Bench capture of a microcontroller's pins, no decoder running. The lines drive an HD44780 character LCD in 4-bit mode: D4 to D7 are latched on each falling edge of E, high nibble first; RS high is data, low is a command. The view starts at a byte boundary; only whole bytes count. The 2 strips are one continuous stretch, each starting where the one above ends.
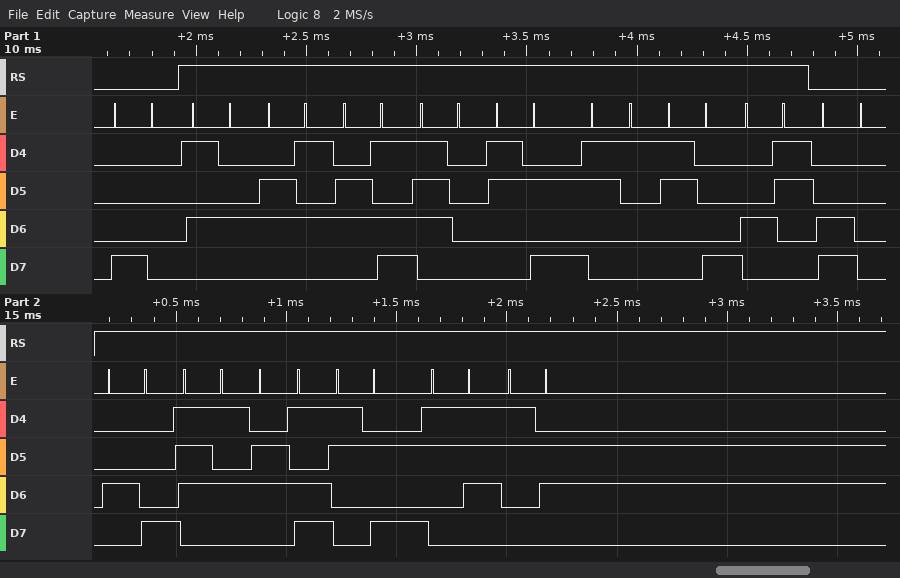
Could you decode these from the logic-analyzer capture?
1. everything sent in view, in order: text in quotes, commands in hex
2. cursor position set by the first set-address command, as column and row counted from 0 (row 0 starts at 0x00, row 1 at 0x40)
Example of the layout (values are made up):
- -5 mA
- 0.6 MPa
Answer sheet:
- 0x80 "Temp:18C" 0xC0 "Hum:76"
- column 0, row 0
